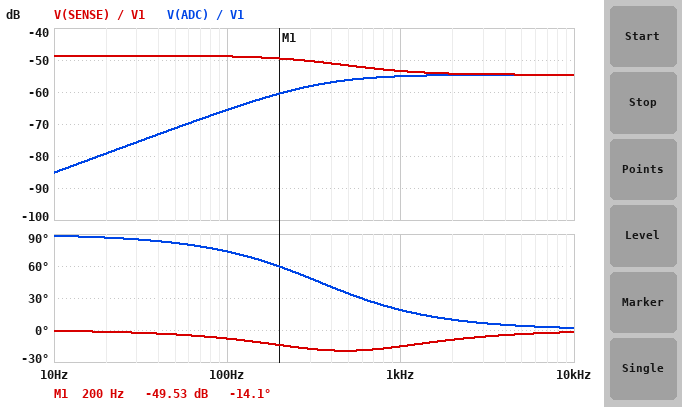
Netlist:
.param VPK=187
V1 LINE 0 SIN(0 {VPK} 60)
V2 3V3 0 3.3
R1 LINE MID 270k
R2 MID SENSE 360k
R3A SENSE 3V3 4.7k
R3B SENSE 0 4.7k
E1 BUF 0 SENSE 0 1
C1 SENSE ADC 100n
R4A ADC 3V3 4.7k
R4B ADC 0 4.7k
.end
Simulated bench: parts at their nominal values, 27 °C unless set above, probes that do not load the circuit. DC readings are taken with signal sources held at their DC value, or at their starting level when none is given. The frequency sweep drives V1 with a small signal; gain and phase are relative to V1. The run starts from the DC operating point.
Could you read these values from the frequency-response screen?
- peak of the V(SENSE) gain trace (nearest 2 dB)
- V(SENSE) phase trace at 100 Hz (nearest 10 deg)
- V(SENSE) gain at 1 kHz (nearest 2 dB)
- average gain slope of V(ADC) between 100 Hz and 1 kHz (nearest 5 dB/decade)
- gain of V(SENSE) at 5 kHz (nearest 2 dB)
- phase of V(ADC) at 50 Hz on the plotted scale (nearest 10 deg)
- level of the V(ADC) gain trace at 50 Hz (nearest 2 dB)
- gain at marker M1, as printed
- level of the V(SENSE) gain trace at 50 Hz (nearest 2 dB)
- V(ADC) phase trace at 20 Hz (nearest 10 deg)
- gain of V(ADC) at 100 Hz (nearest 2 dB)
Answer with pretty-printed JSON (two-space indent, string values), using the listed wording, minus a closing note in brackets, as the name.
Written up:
{
  "peak of the V(SENSE) gain trace": "-48 dB",
  "V(SENSE) phase trace at 100 Hz": "-10 deg",
  "V(SENSE) gain at 1 kHz": "-54 dB",
  "average gain slope of V(ADC) between 100 Hz and 1 kHz": "10 dB/decade",
  "gain of V(SENSE) at 5 kHz": "-54 dB",
  "phase of V(ADC) at 50 Hz on the plotted scale": "80 deg",
  "level of the V(ADC) gain trace at 50 Hz": "-72 dB",
  "gain at marker M1, as printed": "-49.53 dB",
  "level of the V(SENSE) gain trace at 50 Hz": "-48 dB",
  "V(ADC) phase trace at 20 Hz": "90 deg",
  "gain of V(ADC) at 100 Hz": "-66 dB"
}
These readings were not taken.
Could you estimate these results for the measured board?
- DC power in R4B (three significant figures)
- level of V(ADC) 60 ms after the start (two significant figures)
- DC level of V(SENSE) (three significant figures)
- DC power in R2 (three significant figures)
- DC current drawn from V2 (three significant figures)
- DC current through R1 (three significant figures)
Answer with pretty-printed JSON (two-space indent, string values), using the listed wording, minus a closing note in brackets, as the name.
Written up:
{
  "DC power in R4B": "579 µW",
  "level of V(ADC) 60 ms after the start": "1.6 V",
  "DC level of V(SENSE)": "1.64 V",
  "DC power in R2": "2.45 µW",
  "DC current drawn from V2": "703 µA",
  "DC current through R1": "2.61 µA"
}
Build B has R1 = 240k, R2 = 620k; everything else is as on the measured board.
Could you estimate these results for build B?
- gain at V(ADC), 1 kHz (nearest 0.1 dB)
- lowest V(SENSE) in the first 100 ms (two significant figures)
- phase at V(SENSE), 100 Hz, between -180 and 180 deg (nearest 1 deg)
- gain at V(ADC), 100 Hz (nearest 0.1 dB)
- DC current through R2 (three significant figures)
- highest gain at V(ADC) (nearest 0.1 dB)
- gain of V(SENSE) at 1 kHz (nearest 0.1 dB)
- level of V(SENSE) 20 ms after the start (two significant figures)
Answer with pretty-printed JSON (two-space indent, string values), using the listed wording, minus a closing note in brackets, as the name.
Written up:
{
  "gain at V(ADC), 1 kHz": "-57.8 dB",
  "lowest V(SENSE) in the first 100 ms": "1.1 V",
  "phase at V(SENSE), 100 Hz, between -180 and 180 deg": "-8 deg",
  "gain at V(ADC), 100 Hz": "-68.3 dB",
  "DC current through R2": "1.91 µA",
  "highest gain at V(ADC)": "-57.3 dB",
  "gain of V(SENSE) at 1 kHz": "-56.1 dB",
  "level of V(SENSE) 20 ms after the start": "2.1 V"
}
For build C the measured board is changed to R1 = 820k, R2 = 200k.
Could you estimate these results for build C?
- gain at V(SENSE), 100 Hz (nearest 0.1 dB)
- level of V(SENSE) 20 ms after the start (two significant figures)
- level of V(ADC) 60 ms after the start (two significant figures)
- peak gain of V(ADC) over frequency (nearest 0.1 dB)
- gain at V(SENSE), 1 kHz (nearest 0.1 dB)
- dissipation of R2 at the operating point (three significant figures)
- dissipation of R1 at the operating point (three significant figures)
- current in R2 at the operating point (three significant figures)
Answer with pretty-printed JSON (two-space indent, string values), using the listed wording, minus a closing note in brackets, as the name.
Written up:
{
  "gain at V(SENSE), 100 Hz": "-53.0 dB",
  "level of V(SENSE) 20 ms after the start": "2.0 V",
  "level of V(ADC) 60 ms after the start": "1.6 V",
  "peak gain of V(ADC) over frequency": "-58.8 dB",
  "gain at V(SENSE), 1 kHz": "-57.6 dB",
  "dissipation of R2 at the operating point": "521 nW",
  "dissipation of R1 at the operating point": "2.14 µW",
  "current in R2 at the operating point": "1.61 µA"
}
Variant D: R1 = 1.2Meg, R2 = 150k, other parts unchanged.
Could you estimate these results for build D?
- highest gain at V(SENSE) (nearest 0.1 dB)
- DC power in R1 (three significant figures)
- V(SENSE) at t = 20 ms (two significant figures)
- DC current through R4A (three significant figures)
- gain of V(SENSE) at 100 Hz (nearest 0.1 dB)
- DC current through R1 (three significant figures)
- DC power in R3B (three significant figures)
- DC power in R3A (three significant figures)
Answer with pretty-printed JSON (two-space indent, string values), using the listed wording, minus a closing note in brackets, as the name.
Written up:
{
  "highest gain at V(SENSE)": "-55.2 dB",
  "DC power in R1": "1.79 µW",
  "V(SENSE) at t = 20 ms": "1.9 V",
  "DC current through R4A": "351 µA",
  "gain of V(SENSE) at 100 Hz": "-55.5 dB",
  "DC current through R1": "1.22 µA",
  "DC power in R3B": "577 µW",
  "DC power in R3A": "581 µW"
}
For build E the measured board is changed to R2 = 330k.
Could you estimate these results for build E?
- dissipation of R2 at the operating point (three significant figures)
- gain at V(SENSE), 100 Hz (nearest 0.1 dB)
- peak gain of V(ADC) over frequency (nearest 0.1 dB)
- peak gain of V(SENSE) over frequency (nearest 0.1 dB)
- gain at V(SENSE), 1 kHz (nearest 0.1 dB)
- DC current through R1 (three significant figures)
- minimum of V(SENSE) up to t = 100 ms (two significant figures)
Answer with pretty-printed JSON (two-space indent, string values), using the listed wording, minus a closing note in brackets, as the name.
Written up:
{
  "dissipation of R2 at the operating point": "2.48 µW",
  "gain at V(SENSE), 100 Hz": "-48.4 dB",
  "peak gain of V(ADC) over frequency": "-54.2 dB",
  "peak gain of V(SENSE) over frequency": "-48.2 dB",
  "gain at V(SENSE), 1 kHz": "-53.0 dB",
  "DC current through R1": "2.74 µA",
  "minimum of V(SENSE) up to t = 100 ms": "920 mV"
}
